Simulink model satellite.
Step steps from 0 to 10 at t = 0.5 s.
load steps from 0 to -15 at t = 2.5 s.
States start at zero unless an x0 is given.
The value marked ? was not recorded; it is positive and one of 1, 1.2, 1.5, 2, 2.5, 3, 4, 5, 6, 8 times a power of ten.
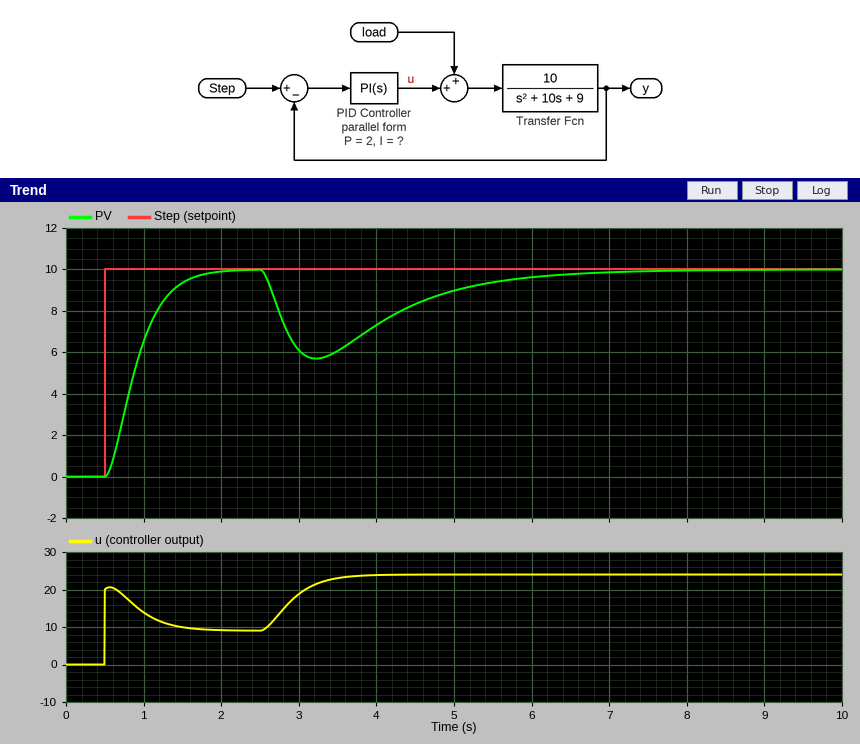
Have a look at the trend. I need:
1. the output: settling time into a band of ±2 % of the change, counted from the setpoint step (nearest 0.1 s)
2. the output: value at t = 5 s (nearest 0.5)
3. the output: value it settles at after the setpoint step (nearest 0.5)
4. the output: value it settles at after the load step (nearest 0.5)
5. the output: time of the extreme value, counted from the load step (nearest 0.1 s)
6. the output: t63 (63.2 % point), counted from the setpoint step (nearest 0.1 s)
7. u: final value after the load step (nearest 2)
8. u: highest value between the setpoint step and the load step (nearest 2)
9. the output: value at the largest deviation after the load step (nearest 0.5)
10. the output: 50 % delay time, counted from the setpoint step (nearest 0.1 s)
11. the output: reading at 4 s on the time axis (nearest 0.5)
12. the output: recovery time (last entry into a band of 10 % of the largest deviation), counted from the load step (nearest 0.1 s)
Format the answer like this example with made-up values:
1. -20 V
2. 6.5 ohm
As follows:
1. 1.3 s
2. 9.0
3. 10.0
4. 10.0
5. 0.7 s
6. 0.5 s
7. 24
8. 20
9. 5.5
10. 0.4 s
11. 7.5
12. 3.4 s
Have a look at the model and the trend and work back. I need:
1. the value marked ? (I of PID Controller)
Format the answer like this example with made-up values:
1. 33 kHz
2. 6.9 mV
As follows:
1. 2
